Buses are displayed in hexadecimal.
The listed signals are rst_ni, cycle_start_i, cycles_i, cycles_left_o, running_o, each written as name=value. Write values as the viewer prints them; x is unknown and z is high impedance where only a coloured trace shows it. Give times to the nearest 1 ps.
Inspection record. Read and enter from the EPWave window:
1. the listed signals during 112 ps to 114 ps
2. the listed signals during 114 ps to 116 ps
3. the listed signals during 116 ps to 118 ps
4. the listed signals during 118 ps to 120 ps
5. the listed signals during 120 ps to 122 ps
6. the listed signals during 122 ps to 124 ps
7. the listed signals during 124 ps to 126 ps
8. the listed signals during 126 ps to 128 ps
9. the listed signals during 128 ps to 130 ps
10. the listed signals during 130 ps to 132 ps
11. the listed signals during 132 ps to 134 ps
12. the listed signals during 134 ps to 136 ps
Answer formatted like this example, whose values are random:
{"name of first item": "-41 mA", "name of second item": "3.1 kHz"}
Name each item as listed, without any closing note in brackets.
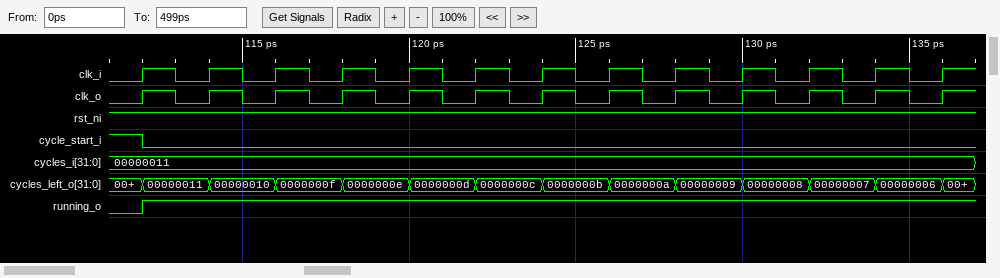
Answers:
{"the listed signals during 112 ps to 114 ps": "rst_ni=1, cycle_start_i=0, cycles_i=00000011, cycles_left_o=00000011, running_o=1", "the listed signals during 114 ps to 116 ps": "rst_ni=1, cycle_start_i=0, cycles_i=00000011, cycles_left_o=00000010, running_o=1", "the listed signals during 116 ps to 118 ps": "rst_ni=1, cycle_start_i=0, cycles_i=00000011, cycles_left_o=0000000f, running_o=1", "the listed signals during 118 ps to 120 ps": "rst_ni=1, cycle_start_i=0, cycles_i=00000011, cycles_left_o=0000000e, running_o=1", "the listed signals during 120 ps to 122 ps": "rst_ni=1, cycle_start_i=0, cycles_i=00000011, cycles_left_o=0000000d, running_o=1", "the listed signals during 122 ps to 124 ps": "rst_ni=1, cycle_start_i=0, cycles_i=00000011, cycles_left_o=0000000c, running_o=1", "the listed signals during 124 ps to 126 ps": "rst_ni=1, cycle_start_i=0, cycles_i=00000011, cycles_left_o=0000000b, running_o=1", "the listed signals during 126 ps to 128 ps": "rst_ni=1, cycle_start_i=0, cycles_i=00000011, cycles_left_o=0000000a, running_o=1", "the listed signals during 128 ps to 130 ps": "rst_ni=1, cycle_start_i=0, cycles_i=00000011, cycles_left_o=00000009, running_o=1", "the listed signals during 130 ps to 132 ps": "rst_ni=1, cycle_start_i=0, cycles_i=00000011, cycles_left_o=00000008, running_o=1", "the listed signals during 132 ps to 134 ps": "rst_ni=1, cycle_start_i=0, cycles_i=00000011, cycles_left_o=00000007, running_o=1", "the listed signals during 134 ps to 136 ps": "rst_ni=1, cycle_start_i=0, cycles_i=00000011, cycles_left_o=00000006, running_o=1"}
